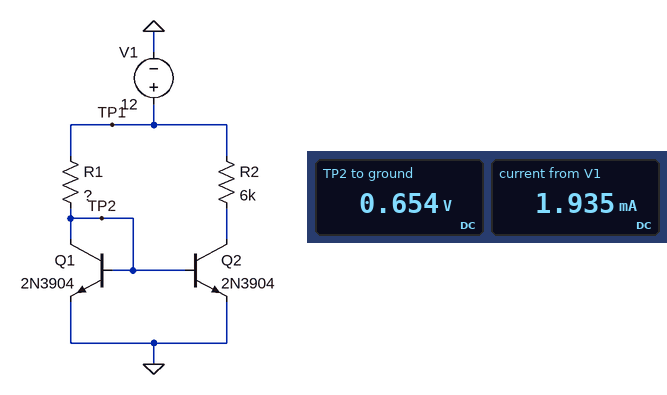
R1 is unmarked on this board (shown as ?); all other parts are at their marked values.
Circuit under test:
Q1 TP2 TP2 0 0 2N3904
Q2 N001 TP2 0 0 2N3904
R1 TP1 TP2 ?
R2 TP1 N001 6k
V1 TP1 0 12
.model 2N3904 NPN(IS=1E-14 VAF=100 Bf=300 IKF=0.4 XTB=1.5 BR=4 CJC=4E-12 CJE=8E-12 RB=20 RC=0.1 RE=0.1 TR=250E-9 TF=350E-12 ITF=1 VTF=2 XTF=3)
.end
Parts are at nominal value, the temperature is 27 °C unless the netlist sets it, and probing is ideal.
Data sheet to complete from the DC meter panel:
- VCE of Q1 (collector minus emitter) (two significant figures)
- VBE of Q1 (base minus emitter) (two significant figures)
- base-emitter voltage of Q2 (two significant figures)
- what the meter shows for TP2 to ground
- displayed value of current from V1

650 mV
650 mV
650 mV
0.654 V
1.935 mA
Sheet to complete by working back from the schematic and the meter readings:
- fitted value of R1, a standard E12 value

12 kΩ
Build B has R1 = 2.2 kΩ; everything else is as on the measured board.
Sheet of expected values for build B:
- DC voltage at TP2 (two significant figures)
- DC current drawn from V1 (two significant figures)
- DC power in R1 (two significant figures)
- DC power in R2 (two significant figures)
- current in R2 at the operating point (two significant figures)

700 mV
7.1 mA
58 mW
24 mW
2.0 mA
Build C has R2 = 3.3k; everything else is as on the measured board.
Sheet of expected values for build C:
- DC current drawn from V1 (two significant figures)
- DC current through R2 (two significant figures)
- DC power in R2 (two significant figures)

2.0 mA
1.0 mA
3.4 mW
